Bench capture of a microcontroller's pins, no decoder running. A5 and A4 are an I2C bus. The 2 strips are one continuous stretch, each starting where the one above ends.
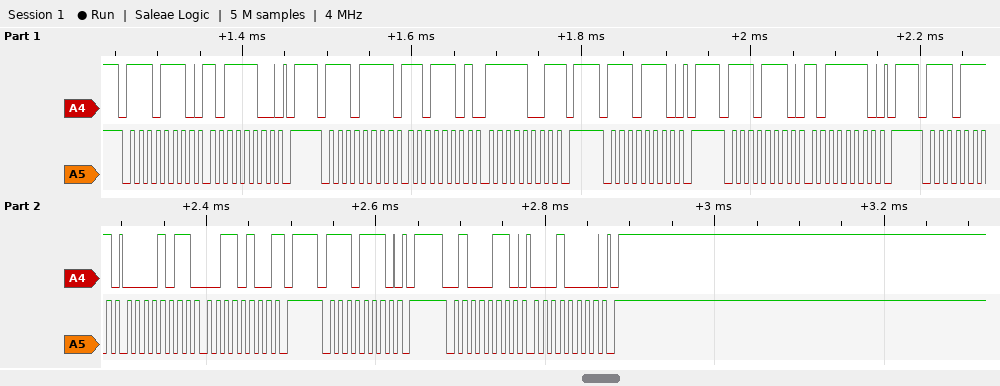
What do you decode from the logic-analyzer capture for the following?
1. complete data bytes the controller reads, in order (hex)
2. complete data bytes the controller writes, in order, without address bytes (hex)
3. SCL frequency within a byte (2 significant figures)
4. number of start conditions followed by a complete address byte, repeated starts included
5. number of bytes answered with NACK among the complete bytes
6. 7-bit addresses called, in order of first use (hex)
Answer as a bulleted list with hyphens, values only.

- DD F9 0B 34
- BC BE 10
- 100 kHz
- 7
- 2
- 0x77 0x23
